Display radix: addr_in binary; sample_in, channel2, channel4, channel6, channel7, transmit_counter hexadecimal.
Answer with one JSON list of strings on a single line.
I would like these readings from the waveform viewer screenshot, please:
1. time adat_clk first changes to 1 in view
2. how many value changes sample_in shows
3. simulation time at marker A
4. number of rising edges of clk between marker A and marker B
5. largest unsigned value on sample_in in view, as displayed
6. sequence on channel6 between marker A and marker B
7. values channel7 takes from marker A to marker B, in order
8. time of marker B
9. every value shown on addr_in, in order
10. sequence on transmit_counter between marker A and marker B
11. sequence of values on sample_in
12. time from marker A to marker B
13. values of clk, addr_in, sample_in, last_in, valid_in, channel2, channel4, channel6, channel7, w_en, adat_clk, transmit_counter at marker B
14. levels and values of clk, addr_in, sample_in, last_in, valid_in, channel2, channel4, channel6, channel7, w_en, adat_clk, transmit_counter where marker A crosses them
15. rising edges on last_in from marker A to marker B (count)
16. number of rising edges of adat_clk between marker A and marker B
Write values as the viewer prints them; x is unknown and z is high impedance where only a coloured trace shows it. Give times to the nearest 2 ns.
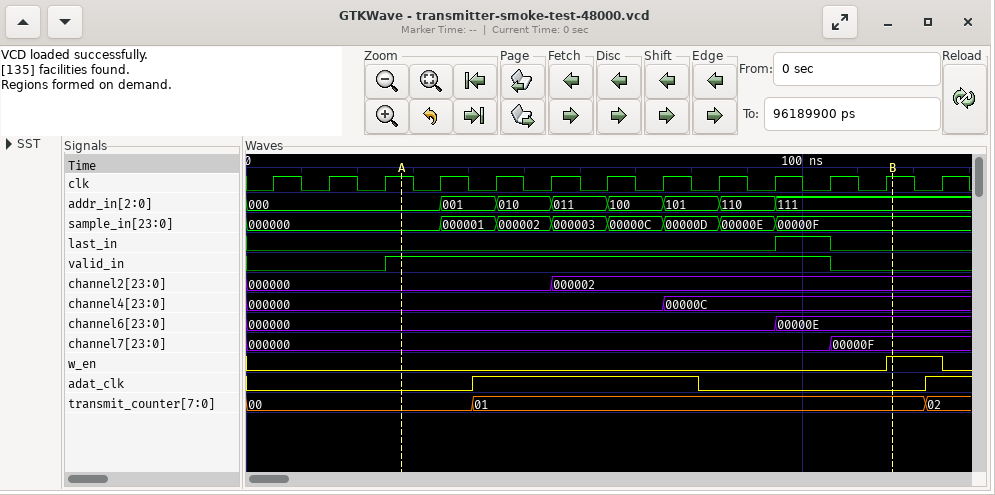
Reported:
["40 ns", "7", "28 ns", "9", "00000F", "000000, 00000E", "000000, 00000F", "116 ns", "000, 001, 010, 011, 100, 101, 110, 111", "00, 01", "000000, 000001, 000002, 000003, 00000C, 00000D, 00000E, 00000F", "88 ns", "clk=1, addr_in=111, sample_in=00000F, last_in=0, valid_in=0, channel2=000002, channel4=00000C, channel6=00000E, channel7=00000F, w_en=1, adat_clk=0, transmit_counter=01", "clk=1, addr_in=000, sample_in=000000, last_in=0, valid_in=1, channel2=000000, channel4=000000, channel6=000000, channel7=000000, w_en=0, adat_clk=0, transmit_counter=00", "1", "1"]
